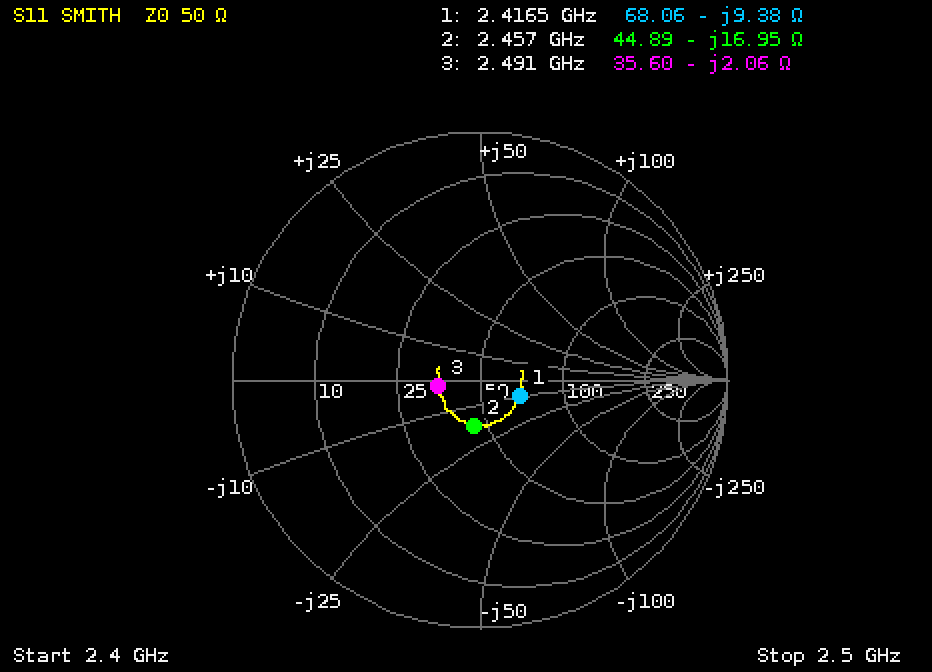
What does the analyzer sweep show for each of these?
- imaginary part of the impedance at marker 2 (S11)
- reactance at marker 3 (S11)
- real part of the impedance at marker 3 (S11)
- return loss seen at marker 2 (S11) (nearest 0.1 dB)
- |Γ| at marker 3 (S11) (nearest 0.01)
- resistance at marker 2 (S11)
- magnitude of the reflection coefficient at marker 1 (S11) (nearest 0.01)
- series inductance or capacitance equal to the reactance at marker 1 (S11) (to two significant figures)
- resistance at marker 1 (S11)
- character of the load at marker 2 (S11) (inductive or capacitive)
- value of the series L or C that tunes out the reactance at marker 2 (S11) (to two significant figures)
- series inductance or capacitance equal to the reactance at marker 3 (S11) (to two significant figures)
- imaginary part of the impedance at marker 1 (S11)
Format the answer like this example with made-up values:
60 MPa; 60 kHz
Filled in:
-16.95 Ω; -2.06 Ω; 35.60 Ω; 14.7 dB; 0.17; 44.89 Ω; 0.17; 7.0 pF; 68.06 Ω; capacitive; 1.1 nH; 31 pF; -9.38 Ω
